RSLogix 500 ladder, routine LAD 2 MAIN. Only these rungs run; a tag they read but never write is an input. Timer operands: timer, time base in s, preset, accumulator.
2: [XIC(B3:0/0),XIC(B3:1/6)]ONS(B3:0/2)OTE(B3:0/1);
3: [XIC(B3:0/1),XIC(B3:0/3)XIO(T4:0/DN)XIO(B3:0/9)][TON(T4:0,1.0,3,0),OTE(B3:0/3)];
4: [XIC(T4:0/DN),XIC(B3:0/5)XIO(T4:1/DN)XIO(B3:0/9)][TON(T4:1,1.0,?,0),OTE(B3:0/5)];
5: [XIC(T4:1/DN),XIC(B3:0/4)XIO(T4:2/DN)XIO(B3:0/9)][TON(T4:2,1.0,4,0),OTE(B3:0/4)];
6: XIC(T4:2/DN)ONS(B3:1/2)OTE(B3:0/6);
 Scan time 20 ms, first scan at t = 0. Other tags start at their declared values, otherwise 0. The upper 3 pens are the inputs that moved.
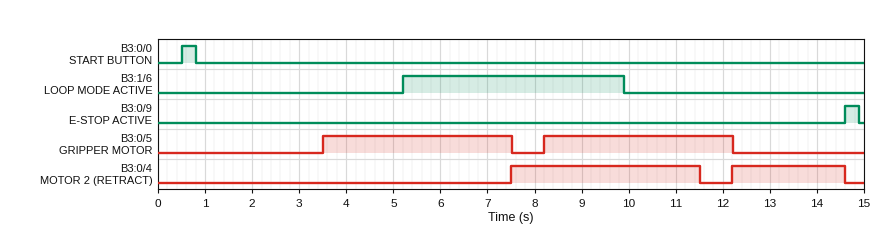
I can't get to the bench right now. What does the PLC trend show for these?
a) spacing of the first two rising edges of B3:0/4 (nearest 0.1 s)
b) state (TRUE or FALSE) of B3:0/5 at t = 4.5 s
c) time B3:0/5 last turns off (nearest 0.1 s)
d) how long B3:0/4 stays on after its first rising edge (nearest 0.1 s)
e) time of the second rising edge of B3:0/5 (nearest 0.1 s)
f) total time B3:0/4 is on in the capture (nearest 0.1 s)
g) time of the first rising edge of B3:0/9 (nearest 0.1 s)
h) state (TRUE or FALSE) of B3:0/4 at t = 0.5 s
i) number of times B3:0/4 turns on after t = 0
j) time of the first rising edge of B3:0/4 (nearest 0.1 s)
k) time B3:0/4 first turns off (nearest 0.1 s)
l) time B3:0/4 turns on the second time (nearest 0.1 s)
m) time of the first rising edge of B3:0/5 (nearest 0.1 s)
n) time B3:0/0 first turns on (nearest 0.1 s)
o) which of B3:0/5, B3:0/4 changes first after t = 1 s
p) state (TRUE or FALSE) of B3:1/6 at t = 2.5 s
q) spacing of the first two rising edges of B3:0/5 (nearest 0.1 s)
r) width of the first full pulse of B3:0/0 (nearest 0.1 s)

4.7 s
TRUE
12.2 s
4.0 s
8.2 s
6.4 s
14.6 s
FALSE
2
7.5 s
11.5 s
12.2 s
3.5 s
0.5 s
B3:0/5
FALSE
4.7 s
0.3 s
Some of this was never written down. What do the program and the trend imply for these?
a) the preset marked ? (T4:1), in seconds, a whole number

4 s
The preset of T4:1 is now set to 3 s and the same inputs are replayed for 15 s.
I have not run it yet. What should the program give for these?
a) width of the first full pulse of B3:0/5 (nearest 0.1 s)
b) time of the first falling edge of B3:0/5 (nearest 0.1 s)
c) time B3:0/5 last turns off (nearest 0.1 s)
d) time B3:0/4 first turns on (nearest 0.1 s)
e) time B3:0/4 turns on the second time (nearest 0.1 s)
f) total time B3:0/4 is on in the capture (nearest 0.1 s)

3.0 s
6.5 s
11.2 s
6.5 s
11.2 s
7.4 s
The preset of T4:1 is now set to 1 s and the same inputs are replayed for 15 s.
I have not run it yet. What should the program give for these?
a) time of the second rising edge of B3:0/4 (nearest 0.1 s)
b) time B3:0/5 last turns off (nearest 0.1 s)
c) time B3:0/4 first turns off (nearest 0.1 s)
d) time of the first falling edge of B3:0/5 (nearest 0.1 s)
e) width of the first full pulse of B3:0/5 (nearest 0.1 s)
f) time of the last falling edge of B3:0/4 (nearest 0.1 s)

9.2 s
9.2 s
8.5 s
4.5 s
1.0 s
13.2 s
